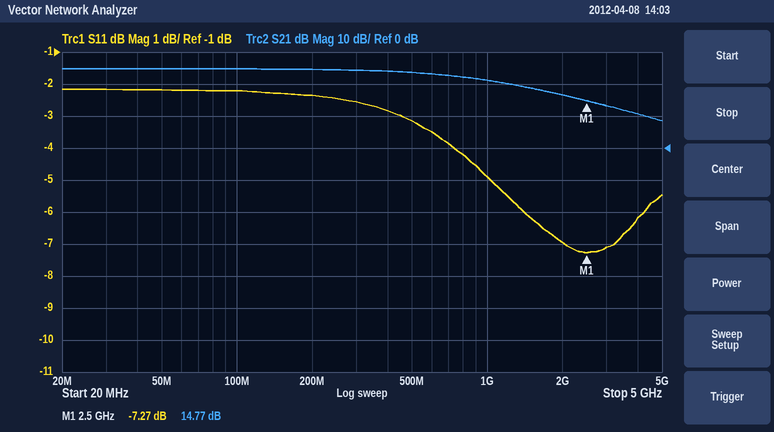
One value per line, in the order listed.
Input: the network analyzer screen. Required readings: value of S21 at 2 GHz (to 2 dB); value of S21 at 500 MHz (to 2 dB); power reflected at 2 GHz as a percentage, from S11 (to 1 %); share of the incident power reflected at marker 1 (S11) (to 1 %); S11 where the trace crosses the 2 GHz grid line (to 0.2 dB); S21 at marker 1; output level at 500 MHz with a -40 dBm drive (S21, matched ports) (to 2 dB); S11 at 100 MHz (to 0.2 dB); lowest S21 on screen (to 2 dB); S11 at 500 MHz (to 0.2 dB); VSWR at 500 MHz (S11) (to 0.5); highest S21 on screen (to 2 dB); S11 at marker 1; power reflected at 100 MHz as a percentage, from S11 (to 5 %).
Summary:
16 dB
24 dB
20 %
19 %
-7.0 dB
14.77 dB
-16 dBm
-2.2 dB
8 dB
-3.2 dB
5.5
24 dB
-7.27 dB
60 %
